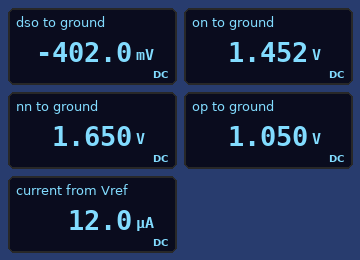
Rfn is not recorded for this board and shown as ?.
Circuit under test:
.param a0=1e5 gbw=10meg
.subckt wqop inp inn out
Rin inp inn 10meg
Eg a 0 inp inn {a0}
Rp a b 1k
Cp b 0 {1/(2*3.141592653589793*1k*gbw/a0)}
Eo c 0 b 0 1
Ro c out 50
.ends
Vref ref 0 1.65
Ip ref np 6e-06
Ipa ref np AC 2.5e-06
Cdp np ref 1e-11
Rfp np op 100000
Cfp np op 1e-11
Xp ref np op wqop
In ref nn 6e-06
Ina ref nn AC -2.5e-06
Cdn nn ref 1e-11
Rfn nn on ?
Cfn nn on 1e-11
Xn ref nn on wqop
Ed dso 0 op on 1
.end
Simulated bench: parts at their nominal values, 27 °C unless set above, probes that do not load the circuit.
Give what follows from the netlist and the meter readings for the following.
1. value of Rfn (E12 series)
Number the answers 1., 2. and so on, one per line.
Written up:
1. 33 kΩ
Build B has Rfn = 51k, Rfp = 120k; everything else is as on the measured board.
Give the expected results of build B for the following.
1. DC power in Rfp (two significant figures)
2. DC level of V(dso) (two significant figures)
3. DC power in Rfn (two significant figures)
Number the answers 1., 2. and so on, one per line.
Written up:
1. 4.3 µW
2. -410 mV
3. 1.8 µW
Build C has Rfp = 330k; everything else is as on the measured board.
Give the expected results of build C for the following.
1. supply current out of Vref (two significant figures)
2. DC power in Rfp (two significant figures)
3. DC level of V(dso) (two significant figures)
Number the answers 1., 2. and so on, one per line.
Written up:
1. 12 µA
2. 12 µW
3. -1.8 V
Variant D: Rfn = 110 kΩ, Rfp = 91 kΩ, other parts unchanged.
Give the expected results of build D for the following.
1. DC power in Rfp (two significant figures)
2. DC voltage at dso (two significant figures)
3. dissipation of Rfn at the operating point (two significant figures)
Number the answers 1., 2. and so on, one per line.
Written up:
1. 3.3 µW
2. 110 mV
3. 4.0 µW
